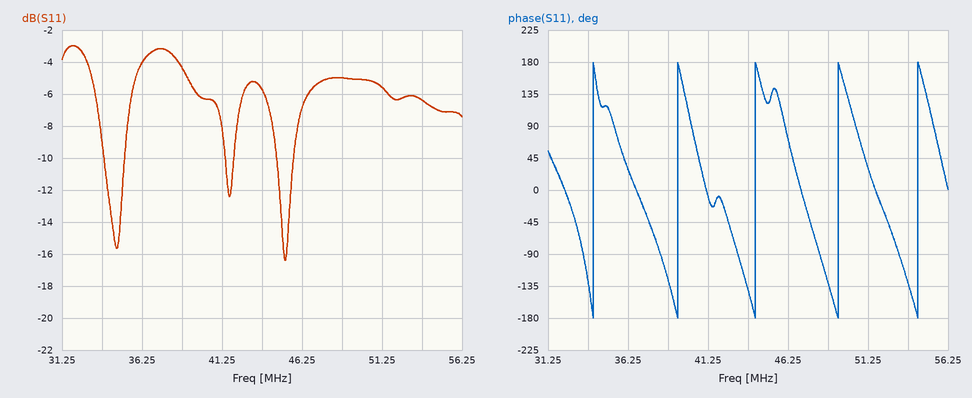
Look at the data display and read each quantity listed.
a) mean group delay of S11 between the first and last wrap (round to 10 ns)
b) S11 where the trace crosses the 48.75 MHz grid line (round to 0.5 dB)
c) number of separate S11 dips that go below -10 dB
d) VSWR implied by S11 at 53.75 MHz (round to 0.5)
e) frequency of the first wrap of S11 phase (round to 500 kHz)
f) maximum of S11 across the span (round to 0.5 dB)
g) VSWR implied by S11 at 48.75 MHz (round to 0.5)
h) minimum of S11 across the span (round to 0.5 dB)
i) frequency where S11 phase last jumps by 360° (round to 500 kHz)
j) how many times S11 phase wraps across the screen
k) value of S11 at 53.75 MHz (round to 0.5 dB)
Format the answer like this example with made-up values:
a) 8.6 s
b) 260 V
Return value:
a) 200 ns
b) -5.0 dB
c) 3
d) 3.0
e) 34.0 MHz
f) -3.0 dB
g) 3.5
h) -16.5 dB
i) 54.5 MHz
j) 5
k) -6.5 dB
